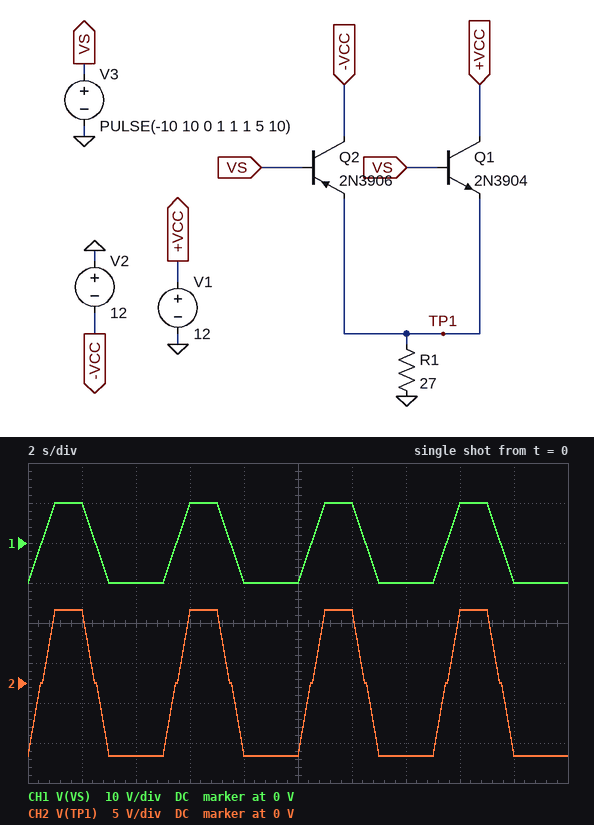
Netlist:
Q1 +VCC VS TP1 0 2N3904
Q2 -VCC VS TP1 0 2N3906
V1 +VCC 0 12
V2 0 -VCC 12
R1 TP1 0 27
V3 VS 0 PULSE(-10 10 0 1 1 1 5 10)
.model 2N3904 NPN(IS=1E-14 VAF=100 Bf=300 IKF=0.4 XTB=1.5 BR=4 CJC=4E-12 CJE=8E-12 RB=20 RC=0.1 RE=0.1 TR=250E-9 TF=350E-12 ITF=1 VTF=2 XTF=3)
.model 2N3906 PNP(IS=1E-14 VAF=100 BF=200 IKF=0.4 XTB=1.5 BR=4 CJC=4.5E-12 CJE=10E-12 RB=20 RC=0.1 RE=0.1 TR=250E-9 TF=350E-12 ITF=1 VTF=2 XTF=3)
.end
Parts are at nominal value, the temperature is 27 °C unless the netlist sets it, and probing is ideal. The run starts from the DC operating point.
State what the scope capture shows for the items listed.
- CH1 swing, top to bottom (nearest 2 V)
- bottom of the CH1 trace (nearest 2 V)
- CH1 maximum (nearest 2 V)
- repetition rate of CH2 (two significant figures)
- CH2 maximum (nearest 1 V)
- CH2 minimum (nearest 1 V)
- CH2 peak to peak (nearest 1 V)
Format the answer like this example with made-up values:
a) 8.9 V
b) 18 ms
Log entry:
a) 20 V
b) -10 V
c) 10 V
d) 200 mHz
e) 9 V
f) -9 V
g) 18 V
